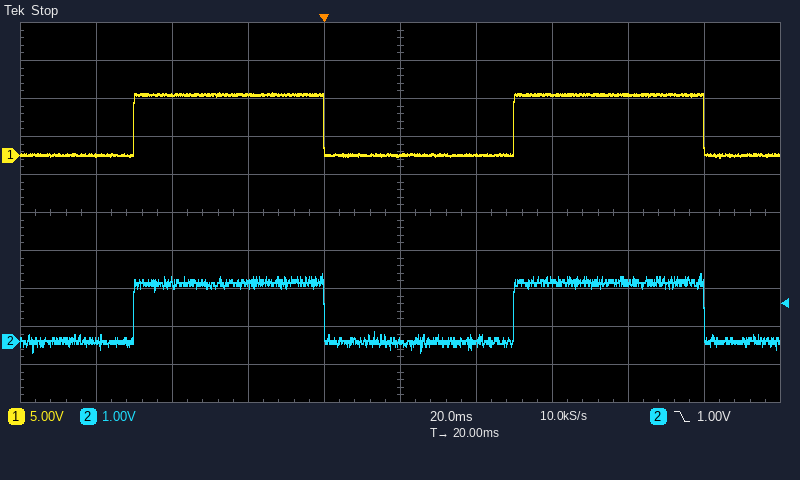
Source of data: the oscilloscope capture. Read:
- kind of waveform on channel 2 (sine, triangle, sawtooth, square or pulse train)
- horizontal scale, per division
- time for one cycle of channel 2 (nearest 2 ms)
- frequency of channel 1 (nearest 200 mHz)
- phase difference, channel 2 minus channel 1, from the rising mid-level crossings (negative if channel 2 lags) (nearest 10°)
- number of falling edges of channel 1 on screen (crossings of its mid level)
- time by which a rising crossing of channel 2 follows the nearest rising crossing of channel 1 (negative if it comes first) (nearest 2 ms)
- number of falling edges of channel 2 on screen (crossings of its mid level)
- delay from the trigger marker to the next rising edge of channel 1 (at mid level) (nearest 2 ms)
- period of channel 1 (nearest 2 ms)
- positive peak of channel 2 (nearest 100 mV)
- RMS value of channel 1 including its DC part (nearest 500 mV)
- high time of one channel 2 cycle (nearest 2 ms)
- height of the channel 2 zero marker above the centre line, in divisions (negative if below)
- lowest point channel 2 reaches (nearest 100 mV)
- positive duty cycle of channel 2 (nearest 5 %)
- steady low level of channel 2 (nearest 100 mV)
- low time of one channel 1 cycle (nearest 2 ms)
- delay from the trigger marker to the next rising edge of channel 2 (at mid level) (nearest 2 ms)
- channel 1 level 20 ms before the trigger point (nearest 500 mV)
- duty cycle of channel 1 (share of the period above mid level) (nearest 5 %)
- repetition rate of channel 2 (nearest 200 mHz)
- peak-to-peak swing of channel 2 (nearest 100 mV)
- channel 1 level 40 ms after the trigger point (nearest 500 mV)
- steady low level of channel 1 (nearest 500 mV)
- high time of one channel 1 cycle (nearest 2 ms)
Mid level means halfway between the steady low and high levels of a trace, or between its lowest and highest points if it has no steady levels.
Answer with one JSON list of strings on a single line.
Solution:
["square", "20 ms", "100 ms", "10.0 Hz", "0°", "2", "0 ms", "2", "50 ms", "100 ms", "1.8 V", "5.5 V", "50 ms", "-3.4 div", "-300 mV", "50 %", "0.0 V", "50 ms", "50 ms", "8.0 V", "50 %", "10.0 Hz", "2.1 V", "0.0 V", "0.0 V", "50 ms"]
